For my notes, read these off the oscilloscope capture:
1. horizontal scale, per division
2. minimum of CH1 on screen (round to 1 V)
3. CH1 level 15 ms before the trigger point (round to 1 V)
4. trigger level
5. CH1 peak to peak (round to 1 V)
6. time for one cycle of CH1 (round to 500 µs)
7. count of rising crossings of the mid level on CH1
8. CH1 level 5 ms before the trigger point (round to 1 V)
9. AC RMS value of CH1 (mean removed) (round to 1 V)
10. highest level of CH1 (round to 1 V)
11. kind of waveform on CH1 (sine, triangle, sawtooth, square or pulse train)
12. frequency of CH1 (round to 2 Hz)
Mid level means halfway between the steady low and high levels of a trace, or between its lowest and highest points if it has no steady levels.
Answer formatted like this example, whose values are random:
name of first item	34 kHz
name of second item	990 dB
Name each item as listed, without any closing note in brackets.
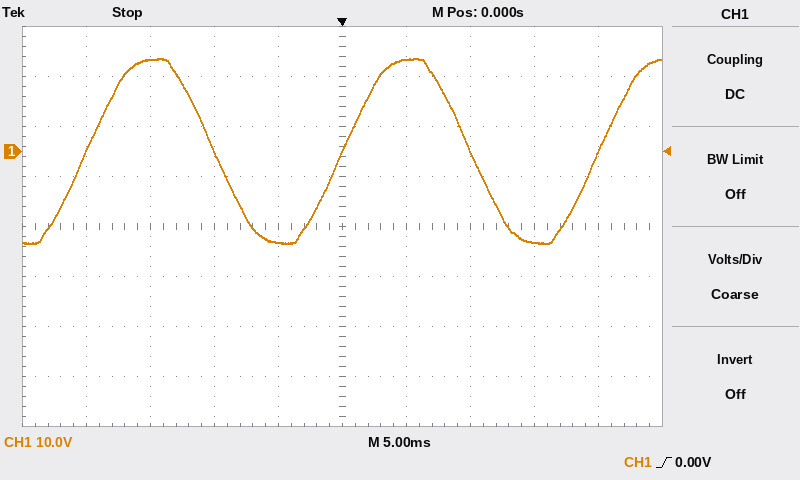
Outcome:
horizontal scale, per division	5 ms
minimum of CH1 on screen	-18 V
CH1 level 15 ms before the trigger point	18 V
trigger level	0.00 V
CH1 peak to peak	37 V
time for one cycle of CH1	20.0 ms
count of rising crossings of the mid level on CH1	3
CH1 level 5 ms before the trigger point	-18 V
AC RMS value of CH1 (mean removed)	13 V
highest level of CH1	19 V
kind of waveform on CH1	sine
frequency of CH1	50 Hz
